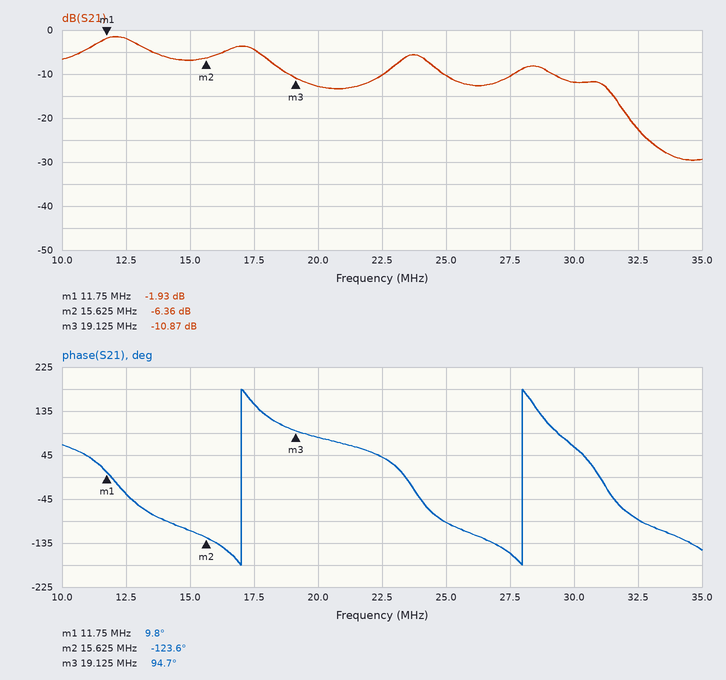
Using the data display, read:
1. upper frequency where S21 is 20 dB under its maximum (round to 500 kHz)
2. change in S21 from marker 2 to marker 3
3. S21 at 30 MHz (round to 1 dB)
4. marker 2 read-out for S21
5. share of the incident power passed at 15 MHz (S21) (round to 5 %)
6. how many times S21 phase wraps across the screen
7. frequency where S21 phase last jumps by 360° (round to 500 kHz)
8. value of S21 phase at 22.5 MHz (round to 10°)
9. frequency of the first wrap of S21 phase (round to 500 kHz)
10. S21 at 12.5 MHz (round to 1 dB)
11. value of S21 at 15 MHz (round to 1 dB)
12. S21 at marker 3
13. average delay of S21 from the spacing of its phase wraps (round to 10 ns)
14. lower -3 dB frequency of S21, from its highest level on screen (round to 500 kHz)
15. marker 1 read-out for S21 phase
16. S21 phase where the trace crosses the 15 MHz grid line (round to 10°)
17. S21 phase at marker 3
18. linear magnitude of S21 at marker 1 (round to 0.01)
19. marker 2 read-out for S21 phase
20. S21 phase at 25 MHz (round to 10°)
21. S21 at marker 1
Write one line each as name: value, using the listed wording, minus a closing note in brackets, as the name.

upper frequency where S21 is 20 dB under its maximum: 32.5 MHz
change in S21 from marker 2 to marker 3: -4.51 dB
S21 at 30 MHz: -12 dB
marker 2 read-out for S21: -6.36 dB
share of the incident power passed at 15 MHz (S21): 20 %
how many times S21 phase wraps across the screen: 2
frequency where S21 phase last jumps by 360°: 28.0 MHz
value of S21 phase at 22.5 MHz: 40°
frequency of the first wrap of S21 phase: 17.0 MHz
S21 at 12.5 MHz: -2 dB
value of S21 at 15 MHz: -7 dB
S21 at marker 3: -10.87 dB
average delay of S21 from the spacing of its phase wraps: 90 ns
lower -3 dB frequency of S21, from its highest level on screen: 11.0 MHz
marker 1 read-out for S21 phase: 9.8°
S21 phase where the trace crosses the 15 MHz grid line: -110°
S21 phase at marker 3: 94.7°
linear magnitude of S21 at marker 1: 0.80
marker 2 read-out for S21 phase: -123.6°
S21 phase at 25 MHz: -90°
S21 at marker 1: -1.93 dB
